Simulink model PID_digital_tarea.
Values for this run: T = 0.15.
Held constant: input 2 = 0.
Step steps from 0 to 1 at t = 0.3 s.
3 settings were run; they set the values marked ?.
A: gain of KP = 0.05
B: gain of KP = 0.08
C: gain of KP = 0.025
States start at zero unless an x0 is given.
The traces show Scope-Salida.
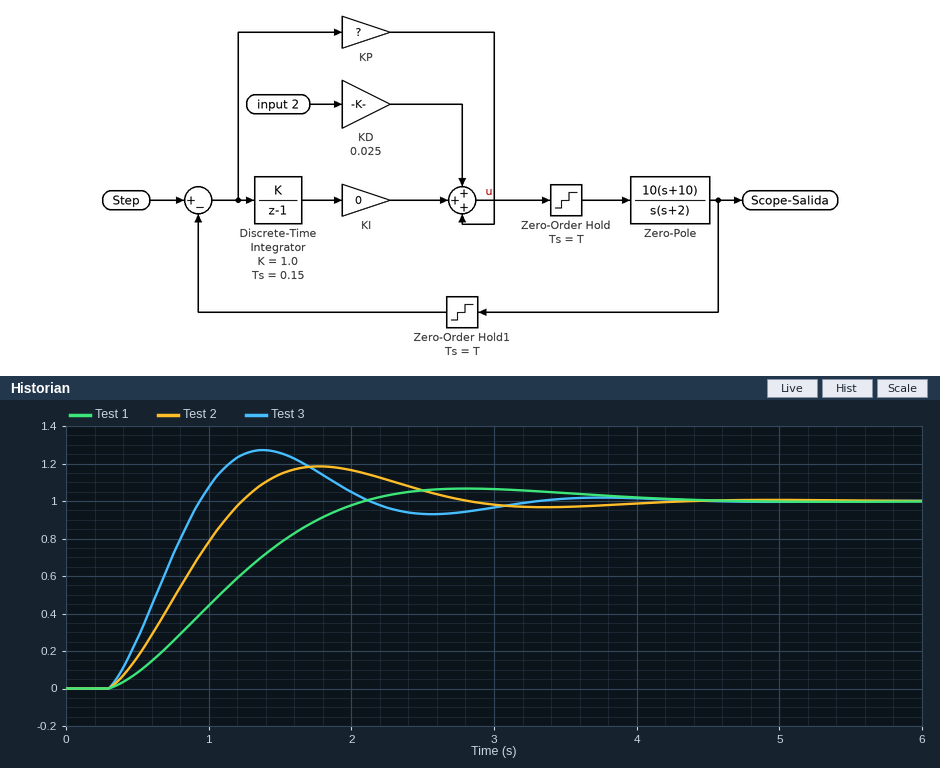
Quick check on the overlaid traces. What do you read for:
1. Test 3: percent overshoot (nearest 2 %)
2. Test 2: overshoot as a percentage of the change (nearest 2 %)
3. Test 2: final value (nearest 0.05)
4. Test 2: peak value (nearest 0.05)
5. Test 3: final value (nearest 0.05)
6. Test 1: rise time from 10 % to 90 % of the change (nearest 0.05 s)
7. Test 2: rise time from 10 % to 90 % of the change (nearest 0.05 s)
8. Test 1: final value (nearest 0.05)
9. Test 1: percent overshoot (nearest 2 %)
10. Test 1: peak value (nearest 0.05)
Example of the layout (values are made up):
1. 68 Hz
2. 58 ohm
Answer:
1. 28 %
2. 18 %
3. 1.00
4. 1.20
5. 1.00
6. 1.25 s
7. 0.70 s
8. 1.00
9. 6 %
10. 1.05
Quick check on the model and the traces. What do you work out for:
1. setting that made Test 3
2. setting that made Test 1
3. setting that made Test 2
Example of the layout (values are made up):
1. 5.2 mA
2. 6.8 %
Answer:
1. B
2. C
3. A
